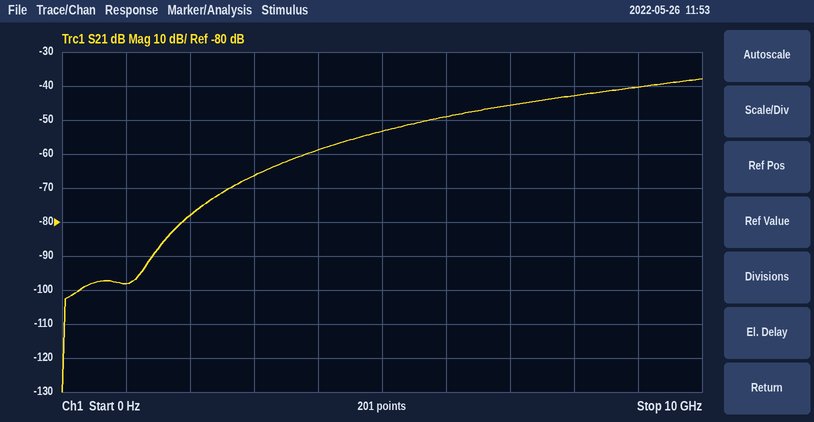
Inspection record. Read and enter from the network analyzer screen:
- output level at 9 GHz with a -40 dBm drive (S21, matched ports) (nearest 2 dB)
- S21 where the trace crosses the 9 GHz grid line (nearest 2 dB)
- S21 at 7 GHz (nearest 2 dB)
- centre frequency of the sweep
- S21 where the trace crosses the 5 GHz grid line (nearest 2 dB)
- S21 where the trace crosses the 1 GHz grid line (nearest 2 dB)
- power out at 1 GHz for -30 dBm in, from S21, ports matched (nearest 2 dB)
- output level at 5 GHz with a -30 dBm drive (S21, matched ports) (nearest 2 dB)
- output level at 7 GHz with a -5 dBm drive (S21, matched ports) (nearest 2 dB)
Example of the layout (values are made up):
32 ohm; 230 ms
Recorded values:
-80 dBm; -40 dB; -46 dB; 5 GHz; -54 dB; -98 dB; -128 dBm; -84 dBm; -50 dBm
